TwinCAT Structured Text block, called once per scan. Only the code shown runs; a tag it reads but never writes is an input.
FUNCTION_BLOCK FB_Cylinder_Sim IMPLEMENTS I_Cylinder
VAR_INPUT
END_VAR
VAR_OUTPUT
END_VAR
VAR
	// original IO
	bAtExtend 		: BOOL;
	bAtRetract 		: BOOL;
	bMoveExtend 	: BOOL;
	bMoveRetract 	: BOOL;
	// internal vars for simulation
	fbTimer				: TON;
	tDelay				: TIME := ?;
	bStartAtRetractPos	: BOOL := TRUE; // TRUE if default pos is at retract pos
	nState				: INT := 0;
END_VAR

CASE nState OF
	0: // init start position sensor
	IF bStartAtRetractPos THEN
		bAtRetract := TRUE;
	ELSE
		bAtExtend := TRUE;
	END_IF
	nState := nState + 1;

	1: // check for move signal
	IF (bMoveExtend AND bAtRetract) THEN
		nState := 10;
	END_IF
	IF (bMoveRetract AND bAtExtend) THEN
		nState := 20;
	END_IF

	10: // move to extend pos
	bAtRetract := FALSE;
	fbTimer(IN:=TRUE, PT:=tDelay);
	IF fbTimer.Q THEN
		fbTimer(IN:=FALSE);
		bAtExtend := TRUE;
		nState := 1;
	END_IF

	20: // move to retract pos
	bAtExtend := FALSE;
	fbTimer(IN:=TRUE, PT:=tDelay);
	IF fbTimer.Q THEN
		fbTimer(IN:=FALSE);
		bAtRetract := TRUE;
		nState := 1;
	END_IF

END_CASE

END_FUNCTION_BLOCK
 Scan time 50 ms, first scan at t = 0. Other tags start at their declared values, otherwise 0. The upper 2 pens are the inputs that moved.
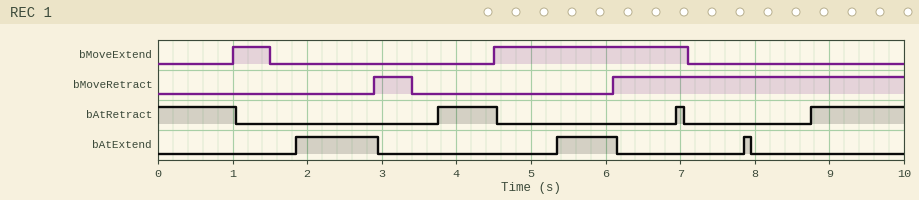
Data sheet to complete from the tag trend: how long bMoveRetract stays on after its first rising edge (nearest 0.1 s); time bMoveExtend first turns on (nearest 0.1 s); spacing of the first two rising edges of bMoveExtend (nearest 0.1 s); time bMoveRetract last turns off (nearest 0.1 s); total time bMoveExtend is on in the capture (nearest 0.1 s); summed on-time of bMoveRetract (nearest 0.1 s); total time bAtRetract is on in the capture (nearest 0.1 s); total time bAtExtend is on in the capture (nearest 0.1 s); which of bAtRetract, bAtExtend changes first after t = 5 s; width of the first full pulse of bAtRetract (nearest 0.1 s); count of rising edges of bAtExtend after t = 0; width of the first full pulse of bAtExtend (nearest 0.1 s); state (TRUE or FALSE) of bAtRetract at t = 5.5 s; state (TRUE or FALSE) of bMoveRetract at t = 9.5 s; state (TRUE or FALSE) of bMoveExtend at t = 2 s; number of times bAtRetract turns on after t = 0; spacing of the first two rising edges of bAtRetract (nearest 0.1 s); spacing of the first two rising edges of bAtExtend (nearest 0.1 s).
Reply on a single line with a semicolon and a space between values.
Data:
0.5 s; 1.0 s; 3.5 s; 3.4 s; 3.1 s; 4.4 s; 3.2 s; 2.0 s; bAtExtend; 0.8 s; 3; 1.1 s; FALSE; TRUE; FALSE; 3; 3.2 s; 3.5 s
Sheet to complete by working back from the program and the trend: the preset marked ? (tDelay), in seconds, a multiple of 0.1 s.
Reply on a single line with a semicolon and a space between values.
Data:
0.8 s
